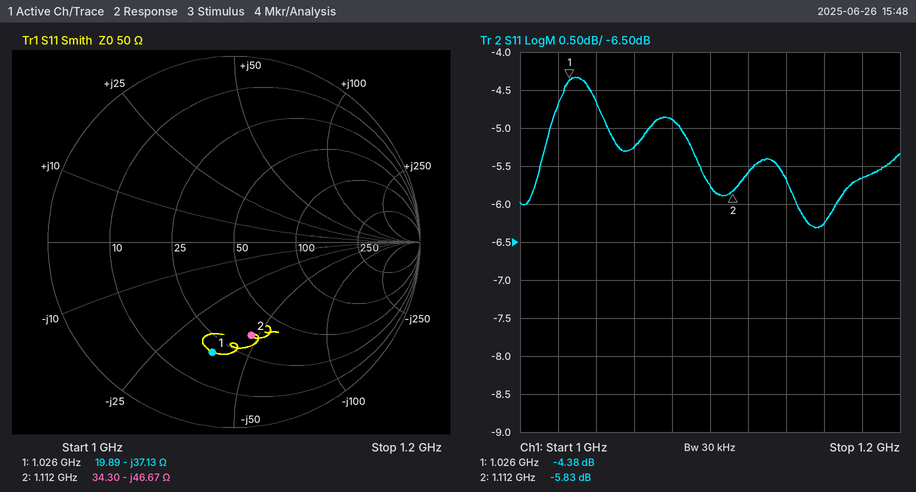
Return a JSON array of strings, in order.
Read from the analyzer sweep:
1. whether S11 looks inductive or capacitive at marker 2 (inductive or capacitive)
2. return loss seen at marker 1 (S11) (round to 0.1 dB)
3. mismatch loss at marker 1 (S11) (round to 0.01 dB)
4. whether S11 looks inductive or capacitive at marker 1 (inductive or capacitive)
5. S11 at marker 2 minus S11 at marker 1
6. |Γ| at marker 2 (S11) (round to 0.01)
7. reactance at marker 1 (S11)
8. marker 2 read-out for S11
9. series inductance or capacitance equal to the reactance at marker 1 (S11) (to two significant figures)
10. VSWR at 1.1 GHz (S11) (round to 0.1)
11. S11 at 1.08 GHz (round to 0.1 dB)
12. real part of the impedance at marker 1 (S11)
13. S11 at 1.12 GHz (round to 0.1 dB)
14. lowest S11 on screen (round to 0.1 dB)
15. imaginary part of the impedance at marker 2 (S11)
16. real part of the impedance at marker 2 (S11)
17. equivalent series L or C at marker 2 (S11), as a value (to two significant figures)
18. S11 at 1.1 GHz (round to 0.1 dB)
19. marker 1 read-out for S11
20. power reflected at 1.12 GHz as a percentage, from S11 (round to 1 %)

["capacitive", "4.4 dB", "1.97 dB", "capacitive", "-1.45 dB", "0.51", "-37.13 Ω", "-5.83 dB", "4.2 pF", "3.1", "-4.9 dB", "19.89 Ω", "-5.6 dB", "-6.3 dB", "-46.67 Ω", "34.30 Ω", "3.1 pF", "-5.8 dB", "-4.38 dB", "28 %"]
